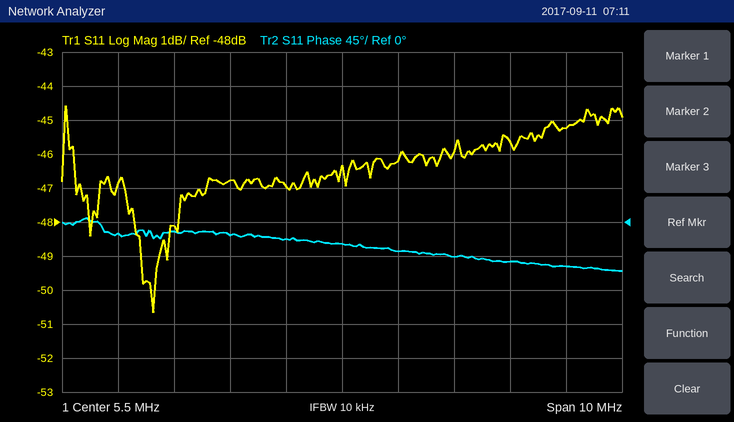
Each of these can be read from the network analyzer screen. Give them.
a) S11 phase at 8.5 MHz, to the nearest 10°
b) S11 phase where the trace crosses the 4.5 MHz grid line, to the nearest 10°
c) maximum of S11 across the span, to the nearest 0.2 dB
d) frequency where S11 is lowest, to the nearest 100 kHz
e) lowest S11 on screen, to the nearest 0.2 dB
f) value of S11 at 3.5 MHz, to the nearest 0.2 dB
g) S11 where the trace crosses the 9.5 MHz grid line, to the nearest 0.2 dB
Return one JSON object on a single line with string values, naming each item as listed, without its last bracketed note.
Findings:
{"S11 phase at 8.5 MHz, to the nearest 10°": "-50°", "S11 phase where the trace crosses the 4.5 MHz grid line, to the nearest 10°": "-20°", "maximum of S11 across the span, to the nearest 0.2 dB": "-44.6 dB", "frequency where S11 is lowest, to the nearest 100 kHz": "2.1 MHz", "lowest S11 on screen, to the nearest 0.2 dB": "-50.6 dB", "value of S11 at 3.5 MHz, to the nearest 0.2 dB": "-46.8 dB", "S11 where the trace crosses the 9.5 MHz grid line, to the nearest 0.2 dB": "-45.2 dB"}
